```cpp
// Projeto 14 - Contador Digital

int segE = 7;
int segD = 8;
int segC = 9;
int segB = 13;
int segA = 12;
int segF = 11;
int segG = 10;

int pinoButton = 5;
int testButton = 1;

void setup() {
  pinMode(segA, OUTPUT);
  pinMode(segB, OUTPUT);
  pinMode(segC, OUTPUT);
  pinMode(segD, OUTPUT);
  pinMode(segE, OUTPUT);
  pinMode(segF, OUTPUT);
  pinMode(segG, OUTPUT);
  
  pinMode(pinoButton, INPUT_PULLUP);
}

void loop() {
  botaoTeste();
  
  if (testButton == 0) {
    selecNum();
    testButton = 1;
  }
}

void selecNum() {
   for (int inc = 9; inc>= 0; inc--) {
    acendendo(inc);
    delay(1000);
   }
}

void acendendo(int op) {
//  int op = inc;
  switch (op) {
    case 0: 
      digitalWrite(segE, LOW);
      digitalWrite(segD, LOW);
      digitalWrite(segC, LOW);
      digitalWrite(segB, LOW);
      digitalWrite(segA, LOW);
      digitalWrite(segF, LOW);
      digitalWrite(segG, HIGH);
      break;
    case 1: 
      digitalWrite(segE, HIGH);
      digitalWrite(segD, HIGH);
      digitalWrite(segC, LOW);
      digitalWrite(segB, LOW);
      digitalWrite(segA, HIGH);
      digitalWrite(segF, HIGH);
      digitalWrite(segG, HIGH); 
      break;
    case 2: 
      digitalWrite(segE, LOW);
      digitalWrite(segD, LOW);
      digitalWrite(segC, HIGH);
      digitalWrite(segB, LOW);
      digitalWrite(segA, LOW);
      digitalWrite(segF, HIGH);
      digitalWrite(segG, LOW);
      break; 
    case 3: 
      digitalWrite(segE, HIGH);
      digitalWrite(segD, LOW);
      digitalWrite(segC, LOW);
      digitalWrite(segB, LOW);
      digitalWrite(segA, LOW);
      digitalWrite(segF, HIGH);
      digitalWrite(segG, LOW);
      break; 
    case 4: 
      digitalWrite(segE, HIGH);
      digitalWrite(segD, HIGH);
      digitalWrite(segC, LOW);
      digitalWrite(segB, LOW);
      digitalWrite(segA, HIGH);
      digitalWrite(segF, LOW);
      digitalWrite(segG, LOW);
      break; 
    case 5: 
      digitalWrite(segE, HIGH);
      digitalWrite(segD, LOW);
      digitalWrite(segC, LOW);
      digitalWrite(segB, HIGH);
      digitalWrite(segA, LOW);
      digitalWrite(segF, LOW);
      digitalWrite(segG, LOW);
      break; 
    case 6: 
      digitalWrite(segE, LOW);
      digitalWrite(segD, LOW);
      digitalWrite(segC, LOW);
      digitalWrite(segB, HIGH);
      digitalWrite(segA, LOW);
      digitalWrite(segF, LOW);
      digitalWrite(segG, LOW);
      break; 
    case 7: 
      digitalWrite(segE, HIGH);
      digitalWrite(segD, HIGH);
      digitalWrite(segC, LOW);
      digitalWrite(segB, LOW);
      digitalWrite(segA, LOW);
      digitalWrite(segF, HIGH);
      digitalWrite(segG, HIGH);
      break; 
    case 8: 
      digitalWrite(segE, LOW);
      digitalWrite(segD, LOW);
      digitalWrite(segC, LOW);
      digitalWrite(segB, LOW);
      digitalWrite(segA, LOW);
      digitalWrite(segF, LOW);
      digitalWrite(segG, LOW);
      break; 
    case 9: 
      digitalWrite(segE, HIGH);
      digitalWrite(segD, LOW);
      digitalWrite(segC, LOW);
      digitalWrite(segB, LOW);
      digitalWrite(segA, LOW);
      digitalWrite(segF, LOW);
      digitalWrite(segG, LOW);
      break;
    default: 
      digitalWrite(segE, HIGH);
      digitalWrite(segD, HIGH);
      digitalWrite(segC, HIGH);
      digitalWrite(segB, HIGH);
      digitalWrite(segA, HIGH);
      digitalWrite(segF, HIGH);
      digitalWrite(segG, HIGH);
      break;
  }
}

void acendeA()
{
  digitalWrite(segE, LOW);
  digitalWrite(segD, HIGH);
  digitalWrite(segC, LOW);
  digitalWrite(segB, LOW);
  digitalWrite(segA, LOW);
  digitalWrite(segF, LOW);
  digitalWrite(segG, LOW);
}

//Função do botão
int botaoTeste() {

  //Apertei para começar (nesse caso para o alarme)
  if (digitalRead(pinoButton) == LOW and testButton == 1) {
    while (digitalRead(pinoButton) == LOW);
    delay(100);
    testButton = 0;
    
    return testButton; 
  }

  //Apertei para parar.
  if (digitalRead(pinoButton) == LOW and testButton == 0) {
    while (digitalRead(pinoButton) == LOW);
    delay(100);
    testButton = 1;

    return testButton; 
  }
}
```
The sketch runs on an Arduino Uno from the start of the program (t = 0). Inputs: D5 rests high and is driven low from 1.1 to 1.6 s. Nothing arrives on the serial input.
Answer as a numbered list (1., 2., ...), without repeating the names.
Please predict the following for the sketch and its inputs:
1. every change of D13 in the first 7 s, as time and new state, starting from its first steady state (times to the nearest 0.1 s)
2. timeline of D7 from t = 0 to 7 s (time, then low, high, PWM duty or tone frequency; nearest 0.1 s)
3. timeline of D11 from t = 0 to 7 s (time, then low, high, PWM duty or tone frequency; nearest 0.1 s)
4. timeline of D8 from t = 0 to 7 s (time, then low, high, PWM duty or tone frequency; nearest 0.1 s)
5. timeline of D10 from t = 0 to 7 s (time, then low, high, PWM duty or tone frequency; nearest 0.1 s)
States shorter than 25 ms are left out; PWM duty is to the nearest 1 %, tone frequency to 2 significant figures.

1. 0 s low; 4.7 s high; 6.7 s low
2. 0 s low; 1.7 s high; 2.7 s low; 3.7 s high; 4.7 s low; 5.7 s high
3. 0 s low; 3.7 s high; 4.7 s low
4. 0 s low; 3.7 s high; 4.7 s low; 6.7 s high
5. 0 s low; 3.7 s high; 4.7 s low
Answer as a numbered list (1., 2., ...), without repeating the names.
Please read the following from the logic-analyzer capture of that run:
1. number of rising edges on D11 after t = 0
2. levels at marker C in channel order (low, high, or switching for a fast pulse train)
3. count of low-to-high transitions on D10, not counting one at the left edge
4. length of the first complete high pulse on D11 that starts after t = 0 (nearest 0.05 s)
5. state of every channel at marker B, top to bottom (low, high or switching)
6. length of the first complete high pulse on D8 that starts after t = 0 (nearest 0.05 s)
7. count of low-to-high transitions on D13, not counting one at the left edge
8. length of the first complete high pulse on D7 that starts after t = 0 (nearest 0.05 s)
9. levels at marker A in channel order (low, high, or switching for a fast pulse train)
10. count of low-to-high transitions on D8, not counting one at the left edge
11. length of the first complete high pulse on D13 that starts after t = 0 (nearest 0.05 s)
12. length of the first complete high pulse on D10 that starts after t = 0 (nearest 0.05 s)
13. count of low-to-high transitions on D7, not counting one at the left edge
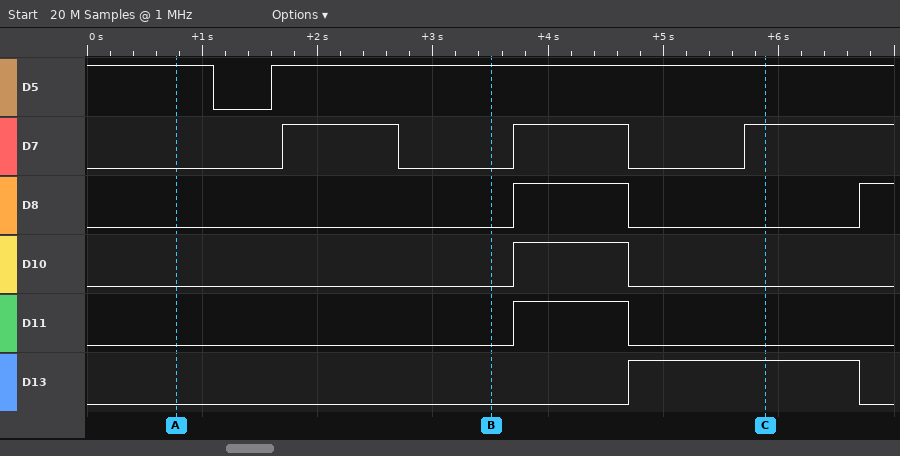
1. 1
2. D5 high, D7 high, D8 low, D10 low, D11 low, D13 high
3. 1
4. 1.00 s
5. D5 high, D7 low, D8 low, D10 low, D11 low, D13 low
6. 1.00 s
7. 1
8. 1.00 s
9. D5 high, D7 low, D8 low, D10 low, D11 low, D13 low
10. 2
11. 2.00 s
12. 1.00 s
13. 3
